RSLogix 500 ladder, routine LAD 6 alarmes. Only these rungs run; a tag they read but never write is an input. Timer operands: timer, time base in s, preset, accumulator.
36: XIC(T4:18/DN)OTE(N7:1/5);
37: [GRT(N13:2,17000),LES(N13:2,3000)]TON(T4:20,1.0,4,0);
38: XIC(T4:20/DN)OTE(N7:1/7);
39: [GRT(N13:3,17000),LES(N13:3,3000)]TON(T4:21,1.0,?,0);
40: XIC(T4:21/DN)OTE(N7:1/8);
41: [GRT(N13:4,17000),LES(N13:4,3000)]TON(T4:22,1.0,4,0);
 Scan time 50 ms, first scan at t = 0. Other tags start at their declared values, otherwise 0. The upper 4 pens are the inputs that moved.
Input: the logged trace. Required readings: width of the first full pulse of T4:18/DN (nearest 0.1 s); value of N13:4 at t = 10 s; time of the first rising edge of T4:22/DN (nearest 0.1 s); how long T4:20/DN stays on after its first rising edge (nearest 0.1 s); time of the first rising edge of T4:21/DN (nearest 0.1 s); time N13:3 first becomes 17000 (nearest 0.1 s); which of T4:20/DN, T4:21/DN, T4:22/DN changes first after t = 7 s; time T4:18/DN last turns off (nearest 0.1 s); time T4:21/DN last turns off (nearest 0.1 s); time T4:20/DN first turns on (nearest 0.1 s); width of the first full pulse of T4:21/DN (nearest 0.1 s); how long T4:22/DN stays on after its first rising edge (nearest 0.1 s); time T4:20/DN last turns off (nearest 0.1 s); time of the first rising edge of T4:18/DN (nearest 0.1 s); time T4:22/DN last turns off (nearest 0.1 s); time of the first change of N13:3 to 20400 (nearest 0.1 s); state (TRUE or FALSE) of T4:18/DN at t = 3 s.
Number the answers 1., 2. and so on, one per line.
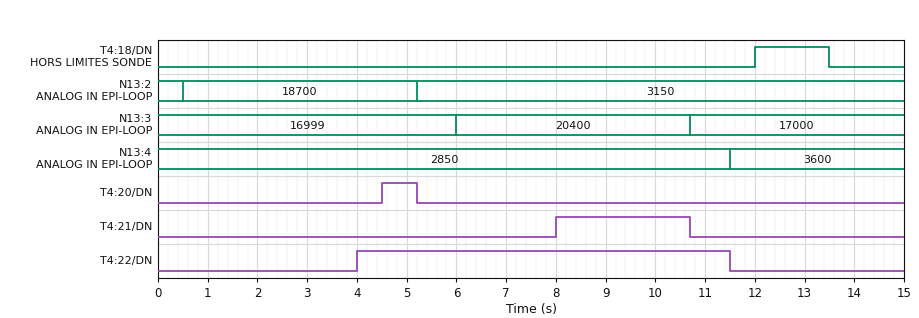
1. 1.5 s
2. 2850
3. 4.0 s
4. 0.7 s
5. 8.0 s
6. 10.7 s
7. T4:21/DN
8. 13.5 s
9. 10.7 s
10. 4.5 s
11. 2.7 s
12. 7.5 s
13. 5.2 s
14. 12.0 s
15. 11.5 s
16. 6.0 s
17. FALSE
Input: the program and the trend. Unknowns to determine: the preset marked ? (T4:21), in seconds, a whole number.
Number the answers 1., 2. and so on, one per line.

1. 2 s
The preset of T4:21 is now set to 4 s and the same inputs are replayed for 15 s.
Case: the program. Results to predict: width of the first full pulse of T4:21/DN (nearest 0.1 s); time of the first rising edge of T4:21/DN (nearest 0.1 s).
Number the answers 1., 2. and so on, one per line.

1. 0.7 s
2. 10.0 s
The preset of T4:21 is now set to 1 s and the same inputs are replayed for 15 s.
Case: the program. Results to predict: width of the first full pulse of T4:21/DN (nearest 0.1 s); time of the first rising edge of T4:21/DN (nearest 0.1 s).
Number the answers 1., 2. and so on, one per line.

1. 3.7 s
2. 7.0 s
